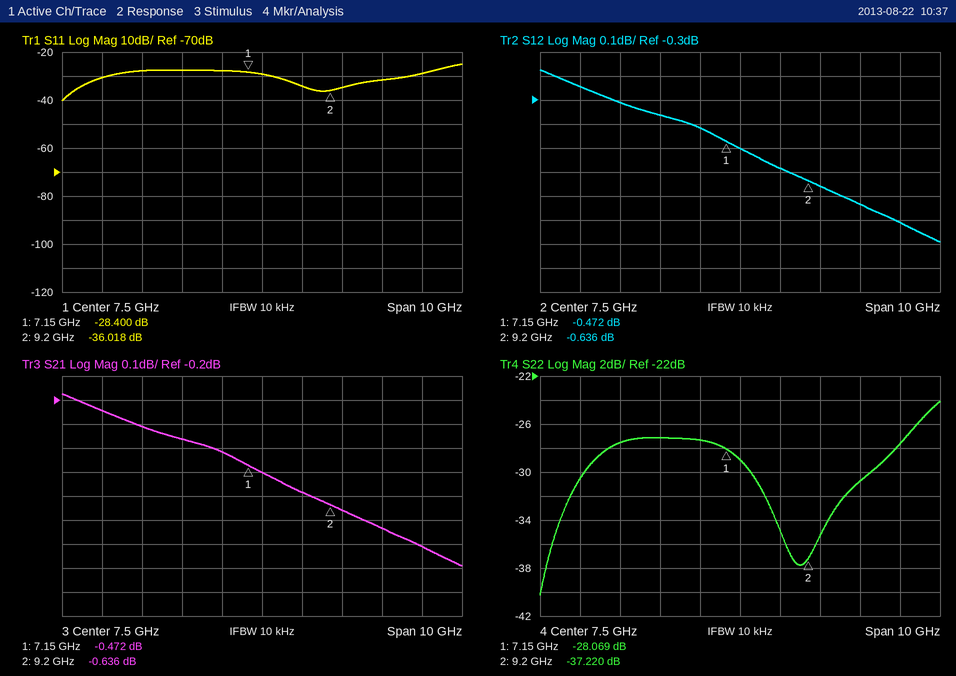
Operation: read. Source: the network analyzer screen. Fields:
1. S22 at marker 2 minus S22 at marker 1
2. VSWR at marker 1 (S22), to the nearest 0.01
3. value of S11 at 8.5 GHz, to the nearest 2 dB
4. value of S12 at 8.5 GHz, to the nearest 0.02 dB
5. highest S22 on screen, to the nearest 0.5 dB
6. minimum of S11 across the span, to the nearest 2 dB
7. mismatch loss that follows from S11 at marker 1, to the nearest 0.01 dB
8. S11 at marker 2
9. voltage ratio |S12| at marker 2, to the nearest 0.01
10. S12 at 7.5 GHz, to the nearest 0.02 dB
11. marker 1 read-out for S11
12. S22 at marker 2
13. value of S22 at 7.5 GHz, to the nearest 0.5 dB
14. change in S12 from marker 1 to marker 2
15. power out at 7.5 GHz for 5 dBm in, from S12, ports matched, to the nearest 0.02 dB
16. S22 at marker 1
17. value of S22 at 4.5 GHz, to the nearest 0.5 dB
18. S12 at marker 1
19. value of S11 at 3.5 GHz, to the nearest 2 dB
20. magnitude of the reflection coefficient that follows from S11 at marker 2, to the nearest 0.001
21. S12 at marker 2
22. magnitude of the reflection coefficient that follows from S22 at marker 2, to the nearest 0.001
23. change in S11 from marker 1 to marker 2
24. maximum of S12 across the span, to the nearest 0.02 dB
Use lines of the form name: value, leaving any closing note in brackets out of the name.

S22 at marker 2 minus S22 at marker 1: -9.151 dB
VSWR at marker 1 (S22), to the nearest 0.01: 1.08
value of S11 at 8.5 GHz, to the nearest 2 dB: -34 dB
value of S12 at 8.5 GHz, to the nearest 0.02 dB: -0.58 dB
highest S22 on screen, to the nearest 0.5 dB: -24.0 dB
minimum of S11 across the span, to the nearest 2 dB: -40 dB
mismatch loss that follows from S11 at marker 1, to the nearest 0.01 dB: 0.01 dB
S11 at marker 2: -36.018 dB
voltage ratio |S12| at marker 2, to the nearest 0.01: 0.93
S12 at 7.5 GHz, to the nearest 0.02 dB: -0.50 dB
marker 1 read-out for S11: -28.400 dB
S22 at marker 2: -37.220 dB
value of S22 at 7.5 GHz, to the nearest 0.5 dB: -29.0 dB
change in S12 from marker 1 to marker 2: -0.164 dB
power out at 7.5 GHz for 5 dBm in, from S12, ports matched, to the nearest 0.02 dB: 4.50 dBm
S22 at marker 1: -28.069 dB
value of S22 at 4.5 GHz, to the nearest 0.5 dB: -27.5 dB
S12 at marker 1: -0.472 dB
value of S11 at 3.5 GHz, to the nearest 2 dB: -30 dB
magnitude of the reflection coefficient that follows from S11 at marker 2, to the nearest 0.001: 0.016
S12 at marker 2: -0.636 dB
magnitude of the reflection coefficient that follows from S22 at marker 2, to the nearest 0.001: 0.014
change in S11 from marker 1 to marker 2: -7.618 dB
maximum of S12 across the span, to the nearest 0.02 dB: -0.18 dB
